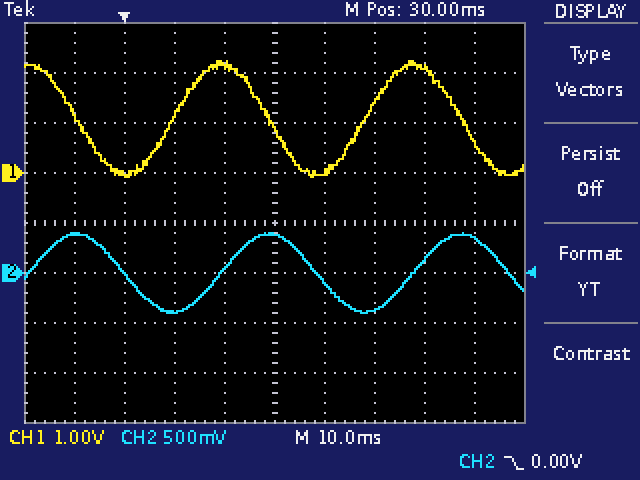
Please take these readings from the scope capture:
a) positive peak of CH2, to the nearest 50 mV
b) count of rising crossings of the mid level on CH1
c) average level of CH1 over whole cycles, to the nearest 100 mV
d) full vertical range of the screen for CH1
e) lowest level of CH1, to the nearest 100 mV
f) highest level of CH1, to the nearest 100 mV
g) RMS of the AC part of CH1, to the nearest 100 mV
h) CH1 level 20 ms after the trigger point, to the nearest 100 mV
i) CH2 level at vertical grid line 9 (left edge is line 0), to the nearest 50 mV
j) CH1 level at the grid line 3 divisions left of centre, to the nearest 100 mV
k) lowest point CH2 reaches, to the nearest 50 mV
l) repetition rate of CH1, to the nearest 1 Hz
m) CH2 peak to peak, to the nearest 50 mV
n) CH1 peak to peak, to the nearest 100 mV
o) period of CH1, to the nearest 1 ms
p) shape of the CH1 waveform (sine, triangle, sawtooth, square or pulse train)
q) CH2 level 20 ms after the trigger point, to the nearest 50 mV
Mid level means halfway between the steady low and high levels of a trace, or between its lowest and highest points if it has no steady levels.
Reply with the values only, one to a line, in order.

400 mV
2
1.1 V
8 V
-100 mV
2.2 V
800 mV
2.2 V
350 mV
0.0 V
-400 mV
26 Hz
800 mV
2.3 V
39 ms
sine
50 mV
